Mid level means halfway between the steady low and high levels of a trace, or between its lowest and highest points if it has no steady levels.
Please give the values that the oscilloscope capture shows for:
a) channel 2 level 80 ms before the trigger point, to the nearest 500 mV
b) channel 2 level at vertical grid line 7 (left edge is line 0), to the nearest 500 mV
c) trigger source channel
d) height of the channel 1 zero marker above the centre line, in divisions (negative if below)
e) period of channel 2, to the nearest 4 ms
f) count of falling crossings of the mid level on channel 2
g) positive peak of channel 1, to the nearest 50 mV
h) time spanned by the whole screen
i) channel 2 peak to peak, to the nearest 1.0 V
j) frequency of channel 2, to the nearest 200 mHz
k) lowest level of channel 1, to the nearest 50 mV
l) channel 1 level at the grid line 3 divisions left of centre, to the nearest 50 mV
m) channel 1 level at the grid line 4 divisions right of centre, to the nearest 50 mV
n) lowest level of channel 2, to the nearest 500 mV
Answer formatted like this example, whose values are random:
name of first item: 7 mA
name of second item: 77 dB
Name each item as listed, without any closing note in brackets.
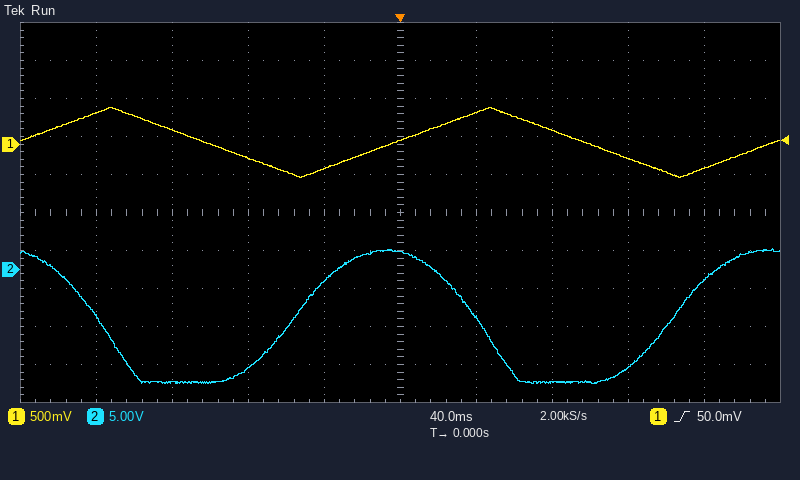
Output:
channel 2 level 80 ms before the trigger point, to the nearest 500 mV: -13.0 V
channel 2 level at vertical grid line 7 (left edge is line 0), to the nearest 500 mV: -15.0 V
trigger source channel: channel 1
height of the channel 1 zero marker above the centre line, in divisions: +1.8 div
period of channel 2, to the nearest 4 ms: 200 ms
count of falling crossings of the mid level on channel 2: 2
positive peak of channel 1, to the nearest 50 mV: 500 mV
time spanned by the whole screen: 400 ms
channel 2 peak to peak, to the nearest 1.0 V: 18.0 V
frequency of channel 2, to the nearest 200 mHz: 5.0 Hz
lowest level of channel 1, to the nearest 50 mV: -450 mV
channel 1 level at the grid line 3 divisions left of centre, to the nearest 50 mV: 200 mV
channel 1 level at the grid line 4 divisions right of centre, to the nearest 50 mV: -300 mV
lowest level of channel 2, to the nearest 500 mV: -15.0 V
